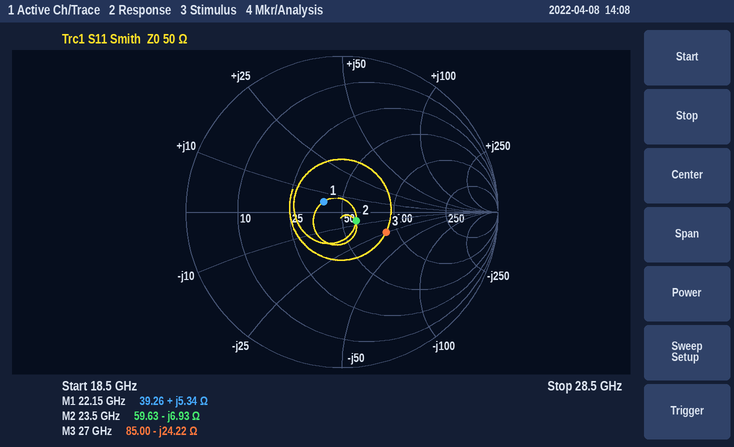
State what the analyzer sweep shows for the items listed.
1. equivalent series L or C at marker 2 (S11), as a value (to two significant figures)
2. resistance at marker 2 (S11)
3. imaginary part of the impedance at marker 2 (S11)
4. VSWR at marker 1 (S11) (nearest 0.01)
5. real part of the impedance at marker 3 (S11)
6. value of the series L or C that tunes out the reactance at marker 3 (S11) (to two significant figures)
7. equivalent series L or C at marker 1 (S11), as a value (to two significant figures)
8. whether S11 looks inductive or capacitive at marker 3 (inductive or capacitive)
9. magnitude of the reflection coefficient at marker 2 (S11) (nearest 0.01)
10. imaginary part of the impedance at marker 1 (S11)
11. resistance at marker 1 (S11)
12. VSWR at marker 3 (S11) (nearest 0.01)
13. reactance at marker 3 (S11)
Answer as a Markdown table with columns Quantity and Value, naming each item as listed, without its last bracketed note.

| Quantity | Value |
|---|---|
| equivalent series L or C at marker 2 (S11), as a value | 980 fF |
| resistance at marker 2 | 59.63 Ω |
| imaginary part of the impedance at marker 2 | -6.93 Ω |
| VSWR at marker 1 (S11) | 1.31 |
| real part of the impedance at marker 3 | 85.00 Ω |
| value of the series L or C that tunes out the reactance at marker 3 (S11) | 140 pH |
| equivalent series L or C at marker 1 (S11), as a value | 38 pH |
| whether S11 looks inductive or capacitive at marker 3 | capacitive |
| magnitude of the reflection coefficient at marker 2 (S11) | 0.11 |
| imaginary part of the impedance at marker 1 | +5.34 Ω |
| resistance at marker 1 | 39.26 Ω |
| VSWR at marker 3 (S11) | 1.90 |
| reactance at marker 3 | -24.22 Ω |
